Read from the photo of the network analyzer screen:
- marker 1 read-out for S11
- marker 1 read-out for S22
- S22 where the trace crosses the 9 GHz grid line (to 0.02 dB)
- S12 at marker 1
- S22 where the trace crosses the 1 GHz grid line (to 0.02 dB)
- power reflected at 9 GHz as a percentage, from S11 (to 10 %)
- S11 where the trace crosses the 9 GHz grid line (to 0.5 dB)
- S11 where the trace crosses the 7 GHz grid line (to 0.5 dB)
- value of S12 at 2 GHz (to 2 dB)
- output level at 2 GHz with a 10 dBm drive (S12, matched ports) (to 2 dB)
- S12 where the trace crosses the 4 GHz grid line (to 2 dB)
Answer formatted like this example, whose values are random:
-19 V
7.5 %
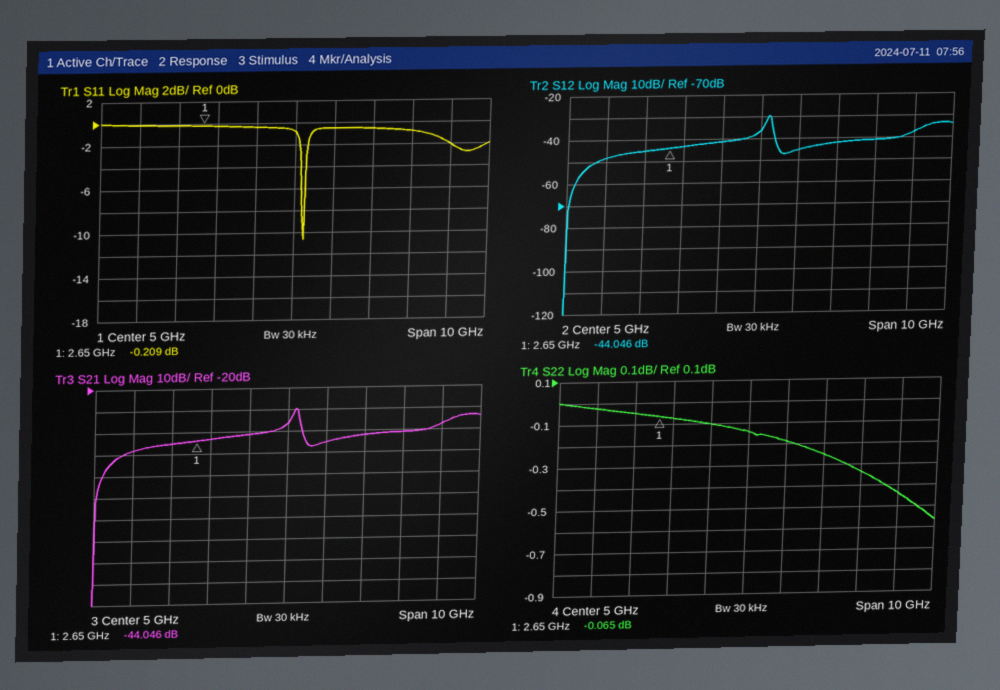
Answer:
-0.209 dB
-0.065 dB
-0.44 dB
-44.046 dB
-0.02 dB
60 %
-2.0 dB
-0.5 dB
-46 dB
-36 dBm
-42 dB
